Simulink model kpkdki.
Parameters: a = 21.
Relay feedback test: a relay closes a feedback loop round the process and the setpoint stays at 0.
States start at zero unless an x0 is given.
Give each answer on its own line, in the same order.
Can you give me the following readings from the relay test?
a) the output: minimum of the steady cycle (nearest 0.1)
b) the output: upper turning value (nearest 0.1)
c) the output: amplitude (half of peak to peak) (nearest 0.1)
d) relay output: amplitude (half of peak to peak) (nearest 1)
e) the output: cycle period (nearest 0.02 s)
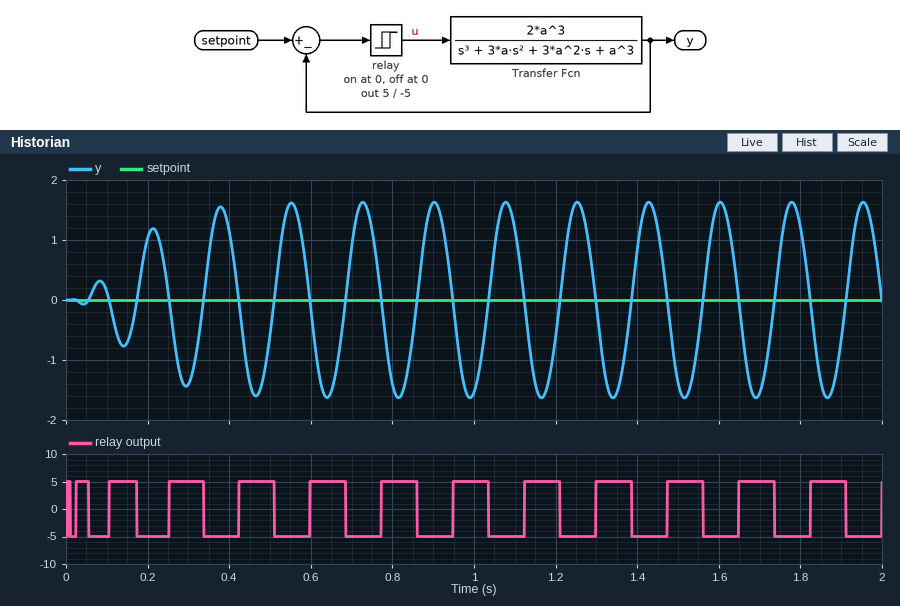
-1.6
1.6
1.6
5
0.18 s
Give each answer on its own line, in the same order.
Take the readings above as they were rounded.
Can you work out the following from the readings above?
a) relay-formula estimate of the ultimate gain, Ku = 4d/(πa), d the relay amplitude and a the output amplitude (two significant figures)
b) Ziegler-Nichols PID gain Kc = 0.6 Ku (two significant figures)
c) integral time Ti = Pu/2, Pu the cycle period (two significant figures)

4.0
2.4
0.090 s
